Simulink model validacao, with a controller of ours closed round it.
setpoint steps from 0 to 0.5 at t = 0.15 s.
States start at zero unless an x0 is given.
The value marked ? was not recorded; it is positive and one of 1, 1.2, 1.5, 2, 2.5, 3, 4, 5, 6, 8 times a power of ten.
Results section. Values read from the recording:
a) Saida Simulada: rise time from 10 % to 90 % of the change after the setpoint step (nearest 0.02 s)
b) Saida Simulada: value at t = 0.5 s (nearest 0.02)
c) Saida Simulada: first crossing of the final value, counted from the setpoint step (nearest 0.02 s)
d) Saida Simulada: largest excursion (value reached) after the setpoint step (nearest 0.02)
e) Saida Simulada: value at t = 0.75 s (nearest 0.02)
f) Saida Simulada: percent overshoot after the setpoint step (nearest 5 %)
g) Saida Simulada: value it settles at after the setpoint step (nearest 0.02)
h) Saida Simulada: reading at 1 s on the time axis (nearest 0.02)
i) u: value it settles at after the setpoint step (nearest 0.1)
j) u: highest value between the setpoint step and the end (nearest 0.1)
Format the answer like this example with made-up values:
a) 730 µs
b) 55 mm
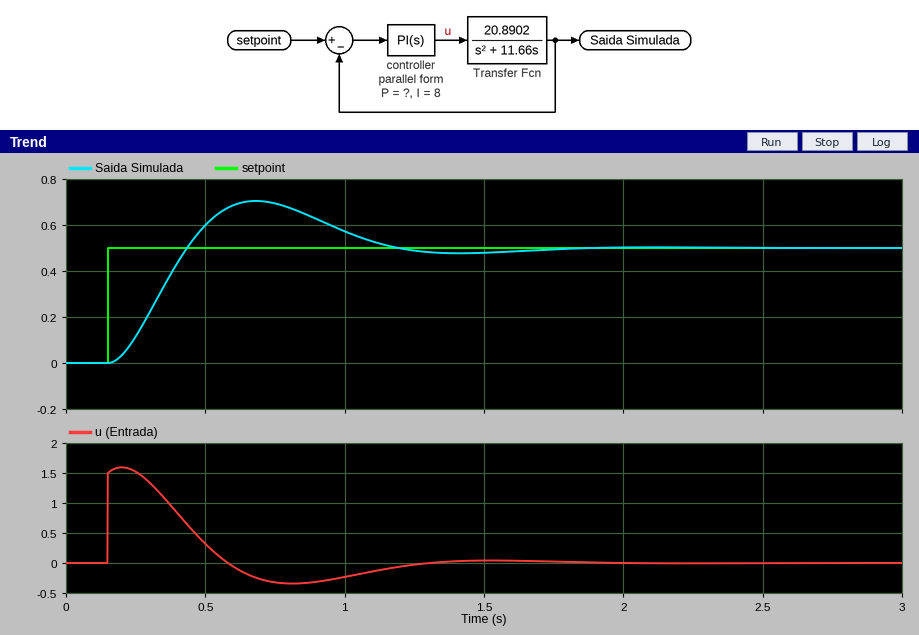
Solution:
a) 0.20 s
b) 0.60
c) 0.28 s
d) 0.70
e) 0.70
f) 40 %
g) 0.50
h) 0.58
i) 0.0
j) 1.6
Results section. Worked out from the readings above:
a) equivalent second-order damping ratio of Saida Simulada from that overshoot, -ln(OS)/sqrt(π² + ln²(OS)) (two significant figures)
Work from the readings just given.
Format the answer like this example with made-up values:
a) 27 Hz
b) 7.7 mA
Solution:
a) 0.28
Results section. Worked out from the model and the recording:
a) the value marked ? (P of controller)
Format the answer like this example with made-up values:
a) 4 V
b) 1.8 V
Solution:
a) 3
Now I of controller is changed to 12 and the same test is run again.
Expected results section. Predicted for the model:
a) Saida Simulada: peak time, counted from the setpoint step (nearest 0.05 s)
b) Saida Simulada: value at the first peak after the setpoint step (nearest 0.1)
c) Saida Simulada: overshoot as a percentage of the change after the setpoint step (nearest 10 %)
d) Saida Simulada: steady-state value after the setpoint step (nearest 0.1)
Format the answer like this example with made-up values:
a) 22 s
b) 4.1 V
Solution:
a) 0.50 s
b) 0.8
c) 50 %
d) 0.5
